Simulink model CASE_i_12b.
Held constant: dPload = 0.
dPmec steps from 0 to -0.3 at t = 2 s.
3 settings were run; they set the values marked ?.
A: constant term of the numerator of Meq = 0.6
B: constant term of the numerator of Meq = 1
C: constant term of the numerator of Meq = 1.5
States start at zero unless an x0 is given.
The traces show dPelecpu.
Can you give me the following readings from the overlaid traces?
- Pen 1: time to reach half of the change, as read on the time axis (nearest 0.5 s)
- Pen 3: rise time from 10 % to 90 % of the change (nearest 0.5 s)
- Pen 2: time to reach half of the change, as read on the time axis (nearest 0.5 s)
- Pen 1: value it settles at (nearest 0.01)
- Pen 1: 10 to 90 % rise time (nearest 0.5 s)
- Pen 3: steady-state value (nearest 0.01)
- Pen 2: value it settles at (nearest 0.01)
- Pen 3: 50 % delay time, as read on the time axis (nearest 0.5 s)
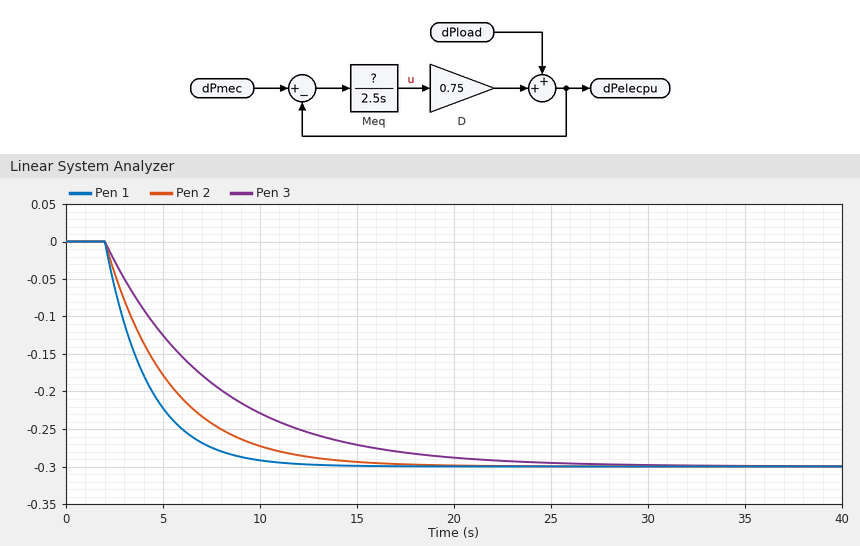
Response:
3.5 s
12.0 s
4.5 s
-0.30
5.0 s
-0.30
-0.30
6.0 s
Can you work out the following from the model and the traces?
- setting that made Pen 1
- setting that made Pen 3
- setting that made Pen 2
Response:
C
A
B
